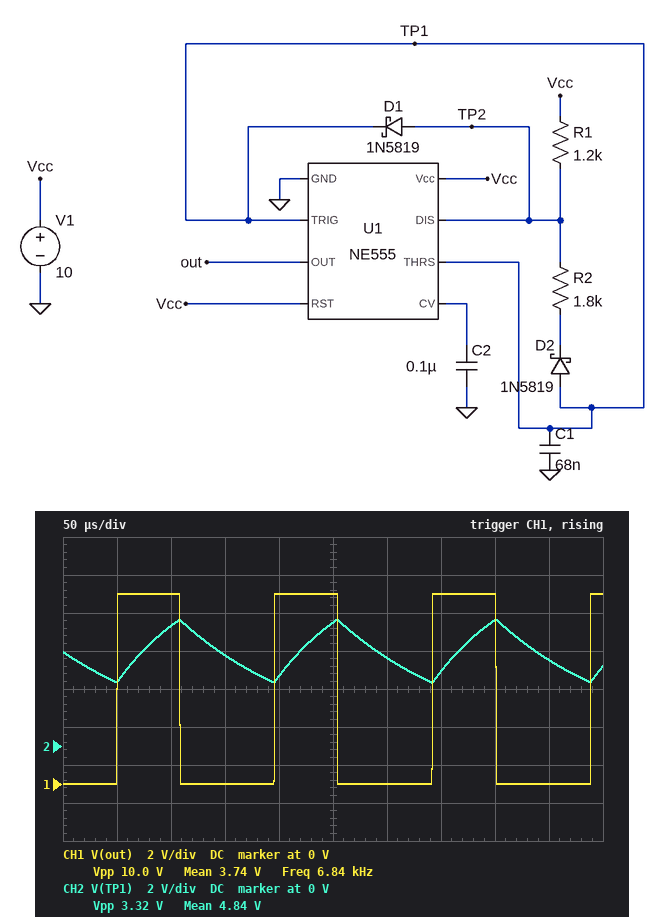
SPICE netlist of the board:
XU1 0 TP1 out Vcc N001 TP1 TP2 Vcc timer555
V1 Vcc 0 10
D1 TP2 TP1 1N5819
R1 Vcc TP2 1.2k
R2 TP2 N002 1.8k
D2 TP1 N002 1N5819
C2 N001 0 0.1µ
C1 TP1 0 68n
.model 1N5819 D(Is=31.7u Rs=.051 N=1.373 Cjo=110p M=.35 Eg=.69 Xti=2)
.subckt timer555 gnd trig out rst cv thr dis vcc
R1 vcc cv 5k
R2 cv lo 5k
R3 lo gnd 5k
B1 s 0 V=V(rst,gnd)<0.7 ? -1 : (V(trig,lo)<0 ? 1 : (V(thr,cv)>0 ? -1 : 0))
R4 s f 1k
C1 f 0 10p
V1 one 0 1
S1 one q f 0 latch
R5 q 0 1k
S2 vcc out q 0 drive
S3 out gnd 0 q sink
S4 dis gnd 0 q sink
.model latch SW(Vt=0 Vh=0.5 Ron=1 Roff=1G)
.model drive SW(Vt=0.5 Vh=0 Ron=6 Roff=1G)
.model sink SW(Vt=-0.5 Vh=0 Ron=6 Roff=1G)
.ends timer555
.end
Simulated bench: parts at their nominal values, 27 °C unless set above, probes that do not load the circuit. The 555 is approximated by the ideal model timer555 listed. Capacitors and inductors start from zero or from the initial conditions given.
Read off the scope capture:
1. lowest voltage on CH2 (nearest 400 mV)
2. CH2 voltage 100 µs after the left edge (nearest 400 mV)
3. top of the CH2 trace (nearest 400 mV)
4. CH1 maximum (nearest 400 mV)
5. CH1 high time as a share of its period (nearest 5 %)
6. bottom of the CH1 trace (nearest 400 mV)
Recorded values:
3.2 V
6.4 V
6.8 V
10.0 V
40 %
0 V
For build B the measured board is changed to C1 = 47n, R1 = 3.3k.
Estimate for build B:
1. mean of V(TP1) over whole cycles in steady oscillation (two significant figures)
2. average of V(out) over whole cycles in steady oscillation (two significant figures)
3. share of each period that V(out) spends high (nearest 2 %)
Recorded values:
5.1 V
6.5 V
64 %
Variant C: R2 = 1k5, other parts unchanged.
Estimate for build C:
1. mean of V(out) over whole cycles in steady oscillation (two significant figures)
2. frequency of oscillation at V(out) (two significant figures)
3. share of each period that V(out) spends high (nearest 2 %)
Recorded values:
4.4 V
7.6 kHz
44 %
